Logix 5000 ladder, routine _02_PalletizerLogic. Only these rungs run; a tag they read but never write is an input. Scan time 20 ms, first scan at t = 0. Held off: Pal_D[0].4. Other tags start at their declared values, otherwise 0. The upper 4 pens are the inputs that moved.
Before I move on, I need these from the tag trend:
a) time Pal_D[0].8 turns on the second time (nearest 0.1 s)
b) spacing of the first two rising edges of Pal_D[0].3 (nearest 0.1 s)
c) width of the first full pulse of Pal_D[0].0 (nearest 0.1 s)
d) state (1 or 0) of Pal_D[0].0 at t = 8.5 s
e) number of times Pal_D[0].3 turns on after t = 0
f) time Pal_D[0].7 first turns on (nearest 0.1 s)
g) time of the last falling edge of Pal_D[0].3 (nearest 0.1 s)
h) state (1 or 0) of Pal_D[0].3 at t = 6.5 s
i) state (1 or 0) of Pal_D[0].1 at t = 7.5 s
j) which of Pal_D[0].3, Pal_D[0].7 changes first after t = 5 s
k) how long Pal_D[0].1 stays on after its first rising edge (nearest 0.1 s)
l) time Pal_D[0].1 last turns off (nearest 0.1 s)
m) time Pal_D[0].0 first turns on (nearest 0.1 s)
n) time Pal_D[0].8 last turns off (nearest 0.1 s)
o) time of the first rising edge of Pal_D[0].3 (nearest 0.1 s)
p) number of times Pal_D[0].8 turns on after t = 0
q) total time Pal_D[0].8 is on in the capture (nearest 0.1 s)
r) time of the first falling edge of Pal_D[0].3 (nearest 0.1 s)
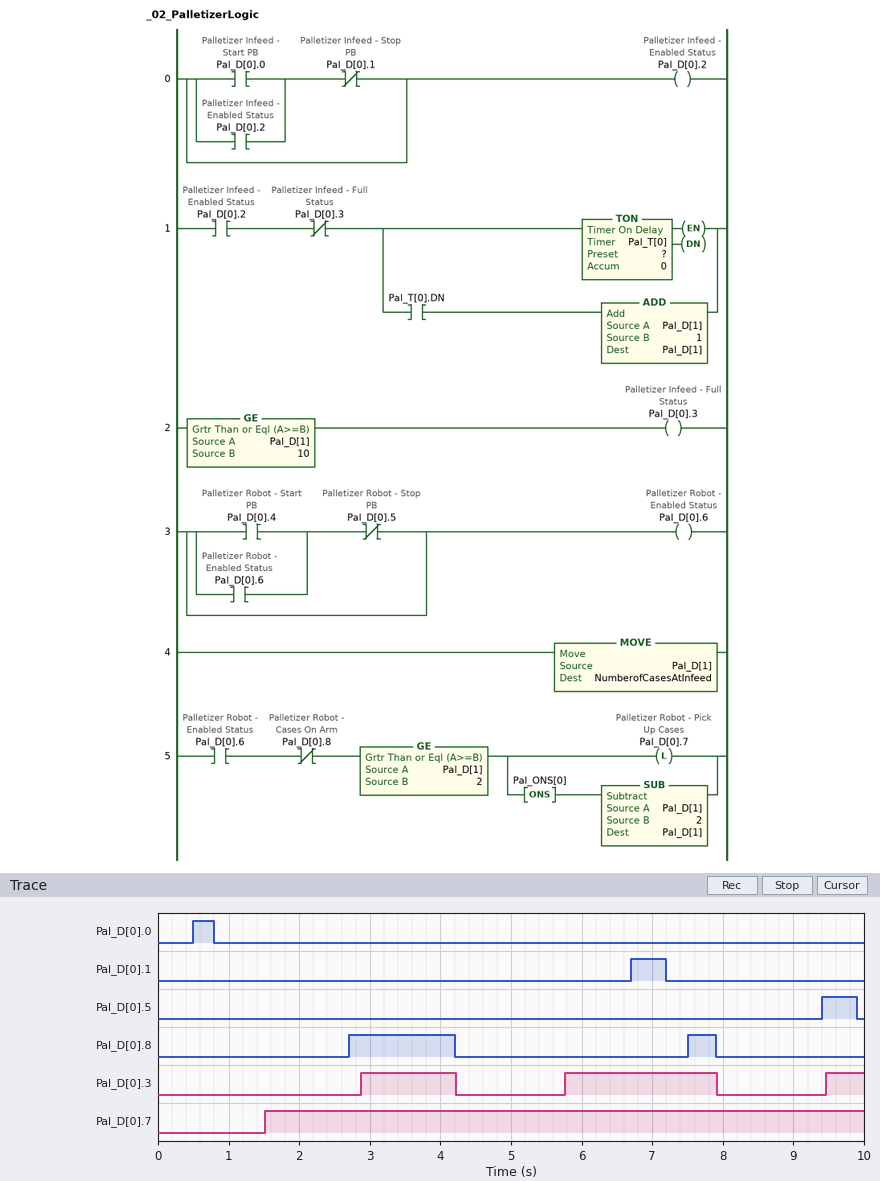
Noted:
7.5 s
2.9 s
0.3 s
0
3
1.5 s
7.9 s
1
0
Pal_D[0].3
0.5 s
7.2 s
0.5 s
7.9 s
2.9 s
2
1.9 s
4.2 s
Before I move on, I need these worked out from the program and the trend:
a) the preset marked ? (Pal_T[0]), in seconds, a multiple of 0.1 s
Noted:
1.5 s
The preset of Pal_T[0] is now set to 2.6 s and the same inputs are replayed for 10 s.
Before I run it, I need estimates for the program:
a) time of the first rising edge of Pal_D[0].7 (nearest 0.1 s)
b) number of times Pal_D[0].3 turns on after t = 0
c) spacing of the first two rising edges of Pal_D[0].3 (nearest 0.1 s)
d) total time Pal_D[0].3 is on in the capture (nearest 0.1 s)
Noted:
2.6 s
2
4.0 s
2.4 s
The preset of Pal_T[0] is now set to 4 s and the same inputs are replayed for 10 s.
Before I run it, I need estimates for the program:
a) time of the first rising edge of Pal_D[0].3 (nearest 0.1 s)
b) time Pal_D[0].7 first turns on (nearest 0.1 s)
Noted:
4.2 s
4.2 s
